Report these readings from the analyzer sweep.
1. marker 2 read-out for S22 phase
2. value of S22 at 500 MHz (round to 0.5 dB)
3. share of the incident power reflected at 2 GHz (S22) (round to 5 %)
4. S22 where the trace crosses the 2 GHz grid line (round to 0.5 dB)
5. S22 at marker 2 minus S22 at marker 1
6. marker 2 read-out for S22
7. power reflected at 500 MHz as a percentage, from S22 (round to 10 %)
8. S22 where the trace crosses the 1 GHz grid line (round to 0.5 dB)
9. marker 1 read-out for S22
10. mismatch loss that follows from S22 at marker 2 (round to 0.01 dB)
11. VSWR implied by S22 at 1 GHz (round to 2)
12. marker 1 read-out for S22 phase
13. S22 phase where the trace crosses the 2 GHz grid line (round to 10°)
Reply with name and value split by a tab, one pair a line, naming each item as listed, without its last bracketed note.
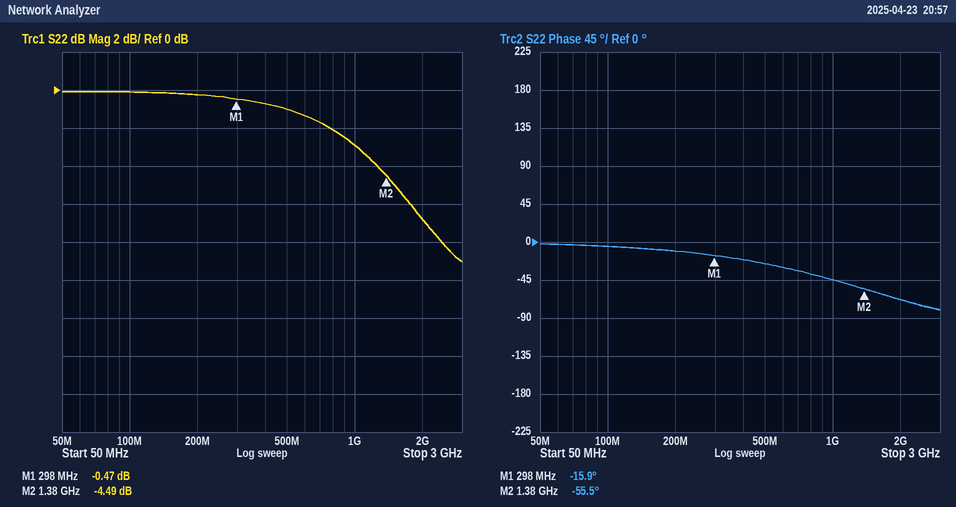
marker 2 read-out for S22 phase	-55.5°
value of S22 at 500 MHz	-1.0 dB
share of the incident power reflected at 2 GHz (S22)	20 %
S22 where the trace crosses the 2 GHz grid line	-7.0 dB
S22 at marker 2 minus S22 at marker 1	-4.02 dB
marker 2 read-out for S22	-4.49 dB
power reflected at 500 MHz as a percentage, from S22	80 %
S22 where the trace crosses the 1 GHz grid line	-3.0 dB
marker 1 read-out for S22	-0.47 dB
mismatch loss that follows from S22 at marker 2	1.91 dB
VSWR implied by S22 at 1 GHz	6
marker 1 read-out for S22 phase	-15.9°
S22 phase where the trace crosses the 2 GHz grid line	-70°
